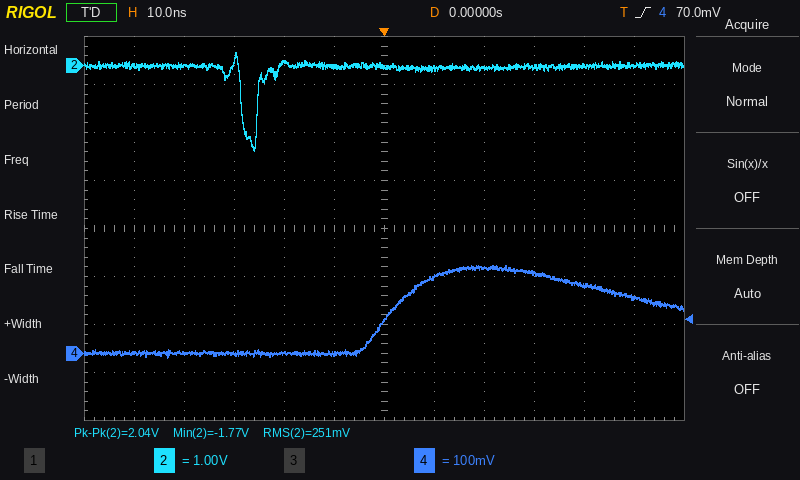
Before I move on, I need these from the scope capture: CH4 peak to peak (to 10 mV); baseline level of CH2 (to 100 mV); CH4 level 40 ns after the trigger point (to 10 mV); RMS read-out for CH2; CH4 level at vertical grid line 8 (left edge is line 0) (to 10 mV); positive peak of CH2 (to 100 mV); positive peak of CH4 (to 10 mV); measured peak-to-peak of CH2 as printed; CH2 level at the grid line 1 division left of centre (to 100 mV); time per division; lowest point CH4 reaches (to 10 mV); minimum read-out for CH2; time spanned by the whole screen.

190 mV
0.0 V
140 mV
251 mV
180 mV
300 mV
180 mV
2.04 V
0.0 V
10 ns
-10 mV
-1.77 V
120 ns
